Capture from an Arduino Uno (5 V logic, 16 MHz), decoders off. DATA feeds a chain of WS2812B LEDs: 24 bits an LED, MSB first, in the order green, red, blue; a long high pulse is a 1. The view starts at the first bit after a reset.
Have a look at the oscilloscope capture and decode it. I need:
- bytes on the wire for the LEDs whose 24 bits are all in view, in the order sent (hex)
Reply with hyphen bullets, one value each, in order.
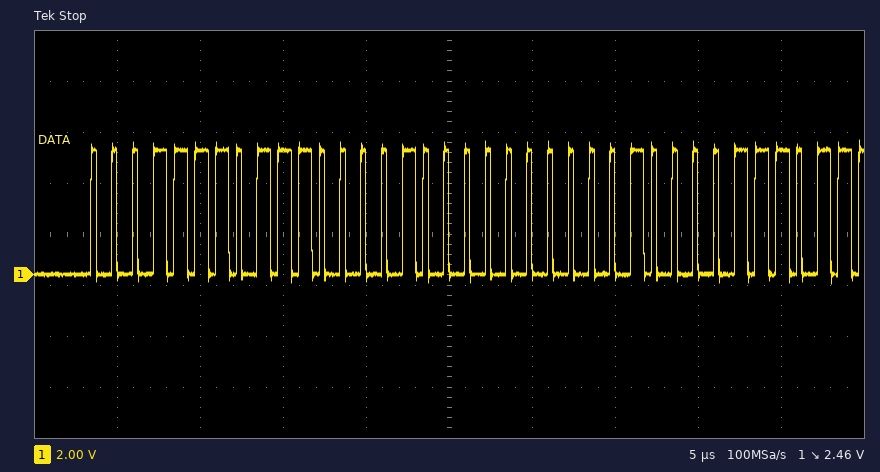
- 1E E1 00
